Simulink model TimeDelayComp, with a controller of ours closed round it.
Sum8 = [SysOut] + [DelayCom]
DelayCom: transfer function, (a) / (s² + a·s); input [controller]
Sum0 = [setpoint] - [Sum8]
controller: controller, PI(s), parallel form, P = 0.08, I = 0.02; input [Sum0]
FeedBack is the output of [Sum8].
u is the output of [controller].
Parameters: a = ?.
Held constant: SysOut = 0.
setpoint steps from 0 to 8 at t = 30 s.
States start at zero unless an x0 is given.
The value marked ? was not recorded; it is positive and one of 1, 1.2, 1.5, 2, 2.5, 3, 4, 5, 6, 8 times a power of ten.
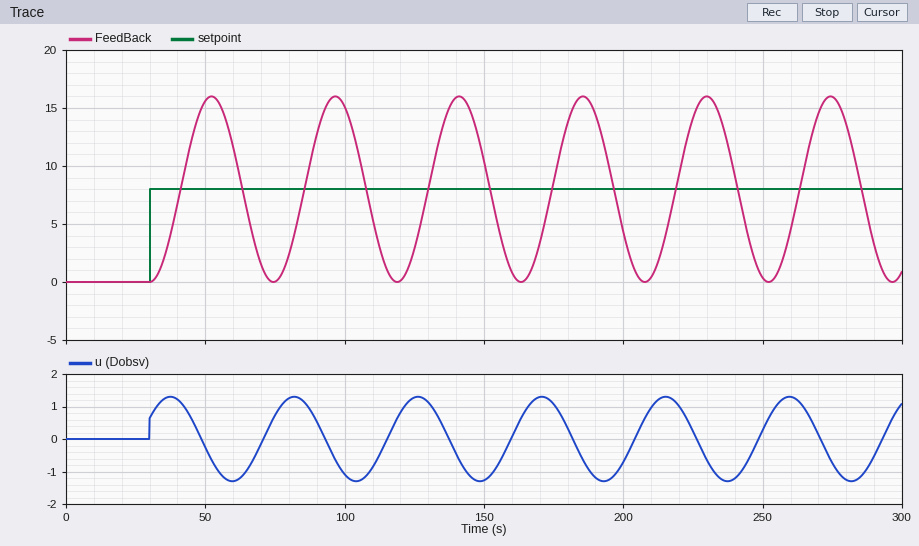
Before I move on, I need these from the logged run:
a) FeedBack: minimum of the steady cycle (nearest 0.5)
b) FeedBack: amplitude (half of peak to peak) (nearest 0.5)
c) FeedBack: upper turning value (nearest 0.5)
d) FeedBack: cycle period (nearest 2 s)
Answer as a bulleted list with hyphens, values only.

- 0.0
- 8.0
- 16.0
- 44 s
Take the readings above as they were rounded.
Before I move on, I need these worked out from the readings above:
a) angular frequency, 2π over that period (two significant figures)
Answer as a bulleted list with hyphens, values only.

- 0.14 rad/s
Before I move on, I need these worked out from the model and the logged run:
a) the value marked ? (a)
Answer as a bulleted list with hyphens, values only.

- 0.25
